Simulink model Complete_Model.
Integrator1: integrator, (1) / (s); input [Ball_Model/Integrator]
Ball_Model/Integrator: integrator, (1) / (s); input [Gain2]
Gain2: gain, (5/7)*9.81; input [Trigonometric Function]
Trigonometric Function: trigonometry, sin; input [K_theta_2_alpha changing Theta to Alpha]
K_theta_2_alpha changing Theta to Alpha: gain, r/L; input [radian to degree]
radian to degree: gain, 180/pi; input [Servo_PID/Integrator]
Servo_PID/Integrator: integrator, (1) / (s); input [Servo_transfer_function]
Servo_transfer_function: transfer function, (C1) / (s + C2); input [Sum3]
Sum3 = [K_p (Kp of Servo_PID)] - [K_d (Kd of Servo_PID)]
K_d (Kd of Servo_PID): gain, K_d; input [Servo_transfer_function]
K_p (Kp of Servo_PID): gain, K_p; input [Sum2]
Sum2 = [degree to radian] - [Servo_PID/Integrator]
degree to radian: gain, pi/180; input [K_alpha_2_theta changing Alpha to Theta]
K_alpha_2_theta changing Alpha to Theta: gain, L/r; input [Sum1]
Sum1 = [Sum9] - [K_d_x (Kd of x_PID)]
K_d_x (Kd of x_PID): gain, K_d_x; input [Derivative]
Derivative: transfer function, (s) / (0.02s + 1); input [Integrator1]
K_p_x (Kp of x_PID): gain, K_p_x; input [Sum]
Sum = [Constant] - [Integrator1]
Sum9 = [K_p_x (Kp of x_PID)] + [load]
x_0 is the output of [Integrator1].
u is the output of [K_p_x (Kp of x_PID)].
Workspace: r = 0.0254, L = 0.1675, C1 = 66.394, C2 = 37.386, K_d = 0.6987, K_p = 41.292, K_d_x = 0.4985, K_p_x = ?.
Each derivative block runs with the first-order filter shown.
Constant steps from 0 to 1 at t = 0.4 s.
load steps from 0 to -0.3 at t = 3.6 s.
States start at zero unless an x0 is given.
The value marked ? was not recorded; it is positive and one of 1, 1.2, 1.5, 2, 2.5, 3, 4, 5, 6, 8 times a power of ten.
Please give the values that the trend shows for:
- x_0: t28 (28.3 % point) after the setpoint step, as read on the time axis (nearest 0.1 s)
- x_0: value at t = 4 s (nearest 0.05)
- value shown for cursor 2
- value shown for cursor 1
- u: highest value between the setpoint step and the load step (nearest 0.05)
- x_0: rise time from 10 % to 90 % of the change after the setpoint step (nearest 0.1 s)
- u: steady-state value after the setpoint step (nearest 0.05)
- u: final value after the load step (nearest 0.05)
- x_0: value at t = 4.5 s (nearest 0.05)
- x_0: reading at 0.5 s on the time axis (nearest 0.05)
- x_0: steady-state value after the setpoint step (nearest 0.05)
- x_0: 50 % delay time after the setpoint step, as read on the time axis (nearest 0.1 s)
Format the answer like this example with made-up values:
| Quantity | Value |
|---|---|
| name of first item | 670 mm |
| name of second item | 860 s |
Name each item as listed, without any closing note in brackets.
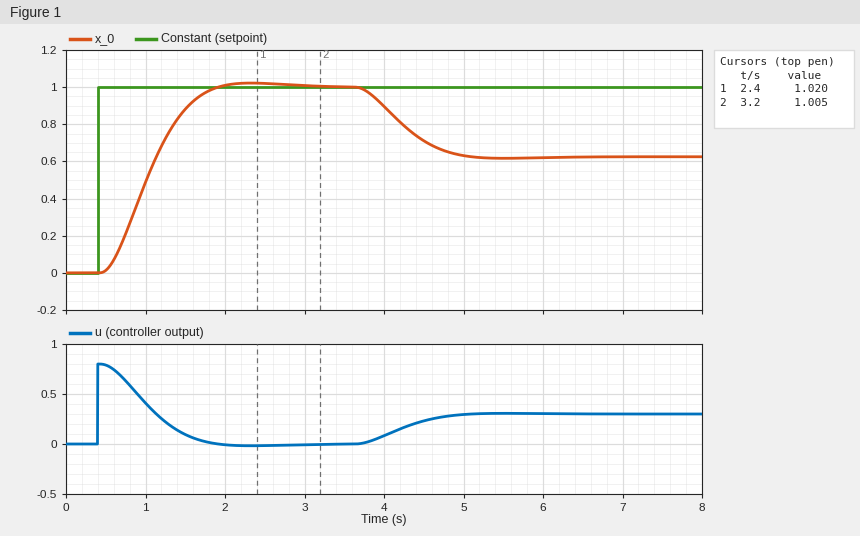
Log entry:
| Quantity | Value |
|---|---|
| x_0: t28 (28.3 % point) after the setpoint step, as read on the time axis | 0.8 s |
| x_0: value at t = 4 s | 0.90 |
| value shown for cursor 2 | 1.005 |
| value shown for cursor 1 | 1.020 |
| u: highest value between the setpoint step and the load step | 0.80 |
| x_0: rise time from 10 % to 90 % of the change after the setpoint step | 0.9 s |
| u: steady-state value after the setpoint step | 0.00 |
| u: final value after the load step | 0.30 |
| x_0: value at t = 4.5 s | 0.70 |
| x_0: reading at 0.5 s on the time axis | 0.00 |
| x_0: steady-state value after the setpoint step | 1.00 |
| x_0: 50 % delay time after the setpoint step, as read on the time axis | 1.0 s |
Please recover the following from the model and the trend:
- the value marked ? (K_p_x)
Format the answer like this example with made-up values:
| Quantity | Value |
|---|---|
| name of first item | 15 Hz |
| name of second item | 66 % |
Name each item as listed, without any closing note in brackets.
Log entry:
| Quantity | Value |
|---|---|
| the value marked ? | 0.8 |
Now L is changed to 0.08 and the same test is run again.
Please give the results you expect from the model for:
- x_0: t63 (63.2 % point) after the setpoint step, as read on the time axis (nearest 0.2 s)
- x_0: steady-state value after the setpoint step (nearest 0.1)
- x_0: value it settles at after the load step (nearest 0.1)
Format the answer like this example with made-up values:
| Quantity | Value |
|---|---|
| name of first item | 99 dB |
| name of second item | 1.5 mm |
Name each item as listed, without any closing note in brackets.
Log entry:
| Quantity | Value |
|---|---|
| x_0: t63 (63.2 % point) after the setpoint step, as read on the time axis | 1.2 s |
| x_0: steady-state value after the setpoint step | 1.0 |
| x_0: value it settles at after the load step | 0.6 |
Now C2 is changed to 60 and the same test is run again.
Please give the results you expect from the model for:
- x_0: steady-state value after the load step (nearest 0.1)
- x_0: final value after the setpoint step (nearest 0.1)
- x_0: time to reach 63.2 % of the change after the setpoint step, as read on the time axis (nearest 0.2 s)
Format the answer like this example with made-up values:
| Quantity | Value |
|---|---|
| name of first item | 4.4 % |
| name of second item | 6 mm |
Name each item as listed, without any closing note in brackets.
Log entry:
| Quantity | Value |
|---|---|
| x_0: steady-state value after the load step | 0.6 |
| x_0: final value after the setpoint step | 1.0 |
| x_0: time to reach 63.2 % of the change after the setpoint step, as read on the time axis | 1.2 s |
